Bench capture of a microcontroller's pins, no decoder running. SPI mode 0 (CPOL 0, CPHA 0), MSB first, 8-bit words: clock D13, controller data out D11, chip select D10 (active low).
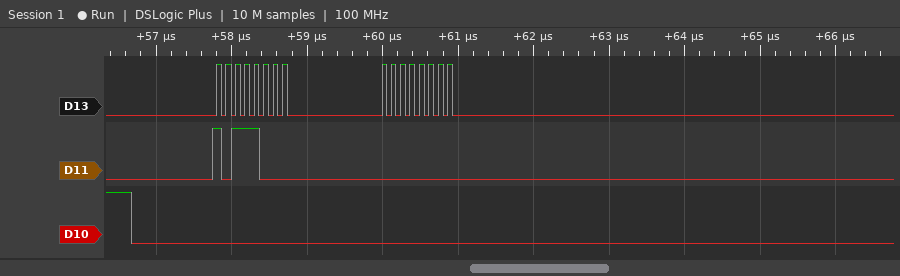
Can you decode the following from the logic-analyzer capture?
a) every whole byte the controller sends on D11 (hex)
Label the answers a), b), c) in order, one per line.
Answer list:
a) 0xB8 0x00
